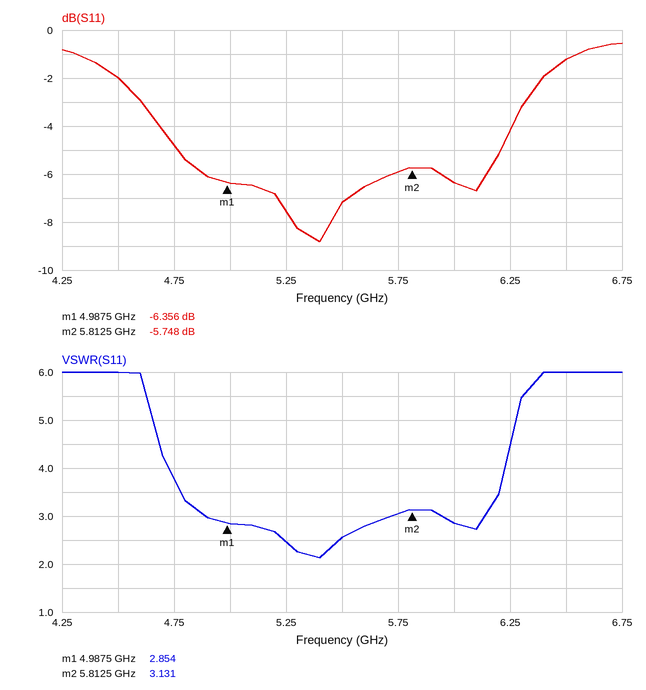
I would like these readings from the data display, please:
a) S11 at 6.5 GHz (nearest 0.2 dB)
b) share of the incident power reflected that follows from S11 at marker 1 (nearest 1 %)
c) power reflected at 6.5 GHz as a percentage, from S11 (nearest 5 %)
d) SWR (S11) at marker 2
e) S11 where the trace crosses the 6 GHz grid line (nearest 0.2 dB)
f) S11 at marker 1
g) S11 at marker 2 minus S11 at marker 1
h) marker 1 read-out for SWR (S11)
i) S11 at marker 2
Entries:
-1.2 dB
23 %
75 %
3.131
-6.4 dB
-6.356 dB
0.608 dB
2.854
-5.748 dB
